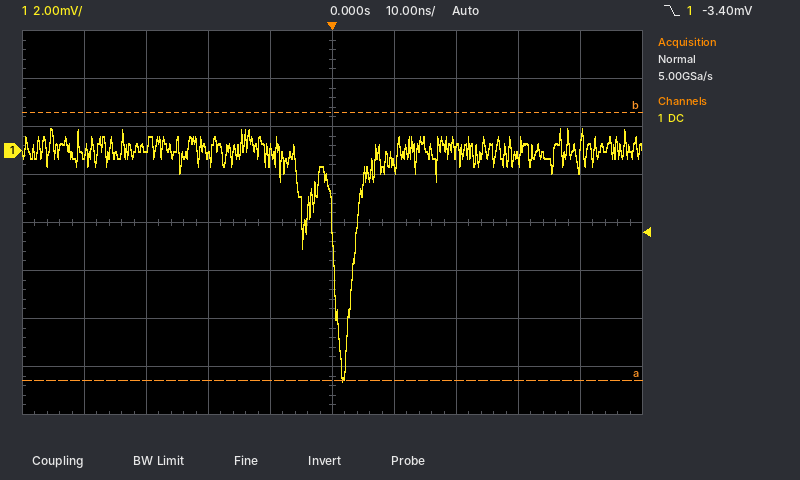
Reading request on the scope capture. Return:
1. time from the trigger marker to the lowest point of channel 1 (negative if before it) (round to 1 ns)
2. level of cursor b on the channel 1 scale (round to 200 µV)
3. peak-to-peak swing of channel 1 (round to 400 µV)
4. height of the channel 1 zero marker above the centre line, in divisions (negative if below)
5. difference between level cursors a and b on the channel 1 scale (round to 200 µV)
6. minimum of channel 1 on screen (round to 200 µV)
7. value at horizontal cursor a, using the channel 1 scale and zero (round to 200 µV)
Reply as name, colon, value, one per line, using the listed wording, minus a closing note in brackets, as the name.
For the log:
time from the trigger marker to the lowest point of channel 1 (negative if before it): +2 ns
level of cursor b on the channel 1 scale: 1.6 mV
peak-to-peak swing of channel 1: 10.4 mV
height of the channel 1 zero marker above the centre line, in divisions: +1.5 div
difference between level cursors a and b on the channel 1 scale: 11.2 mV
minimum of channel 1 on screen: -9.6 mV
value at horizontal cursor a, using the channel 1 scale and zero: -9.6 mV
